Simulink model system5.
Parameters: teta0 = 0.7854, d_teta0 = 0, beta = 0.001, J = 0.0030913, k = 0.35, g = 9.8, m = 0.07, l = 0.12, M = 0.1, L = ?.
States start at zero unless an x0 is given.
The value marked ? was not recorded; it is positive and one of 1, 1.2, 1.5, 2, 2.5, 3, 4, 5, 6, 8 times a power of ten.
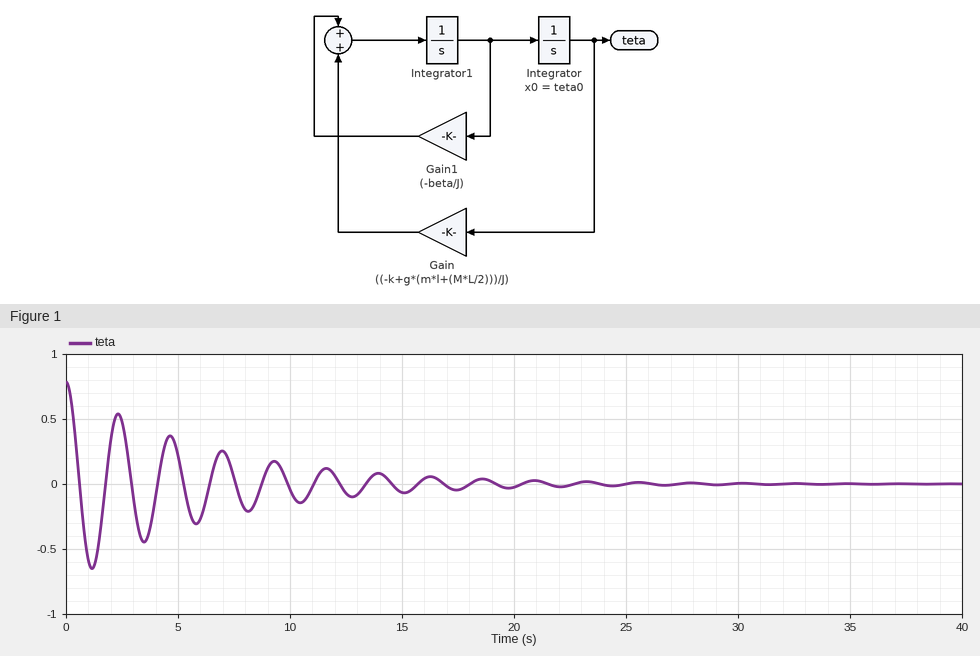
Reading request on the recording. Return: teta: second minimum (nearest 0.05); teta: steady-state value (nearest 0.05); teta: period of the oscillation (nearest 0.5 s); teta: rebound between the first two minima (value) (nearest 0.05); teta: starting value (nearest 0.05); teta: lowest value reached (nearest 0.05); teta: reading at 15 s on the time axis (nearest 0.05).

-0.45
0.00
2.5 s
0.55
0.80
-0.65
-0.05
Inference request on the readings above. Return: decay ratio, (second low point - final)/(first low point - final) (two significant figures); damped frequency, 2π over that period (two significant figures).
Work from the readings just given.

0.69
2.5 rad/s
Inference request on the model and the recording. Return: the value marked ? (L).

0.5
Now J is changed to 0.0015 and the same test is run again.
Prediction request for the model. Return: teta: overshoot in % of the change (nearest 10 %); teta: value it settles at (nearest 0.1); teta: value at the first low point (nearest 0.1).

80 %
0.0
-0.6
